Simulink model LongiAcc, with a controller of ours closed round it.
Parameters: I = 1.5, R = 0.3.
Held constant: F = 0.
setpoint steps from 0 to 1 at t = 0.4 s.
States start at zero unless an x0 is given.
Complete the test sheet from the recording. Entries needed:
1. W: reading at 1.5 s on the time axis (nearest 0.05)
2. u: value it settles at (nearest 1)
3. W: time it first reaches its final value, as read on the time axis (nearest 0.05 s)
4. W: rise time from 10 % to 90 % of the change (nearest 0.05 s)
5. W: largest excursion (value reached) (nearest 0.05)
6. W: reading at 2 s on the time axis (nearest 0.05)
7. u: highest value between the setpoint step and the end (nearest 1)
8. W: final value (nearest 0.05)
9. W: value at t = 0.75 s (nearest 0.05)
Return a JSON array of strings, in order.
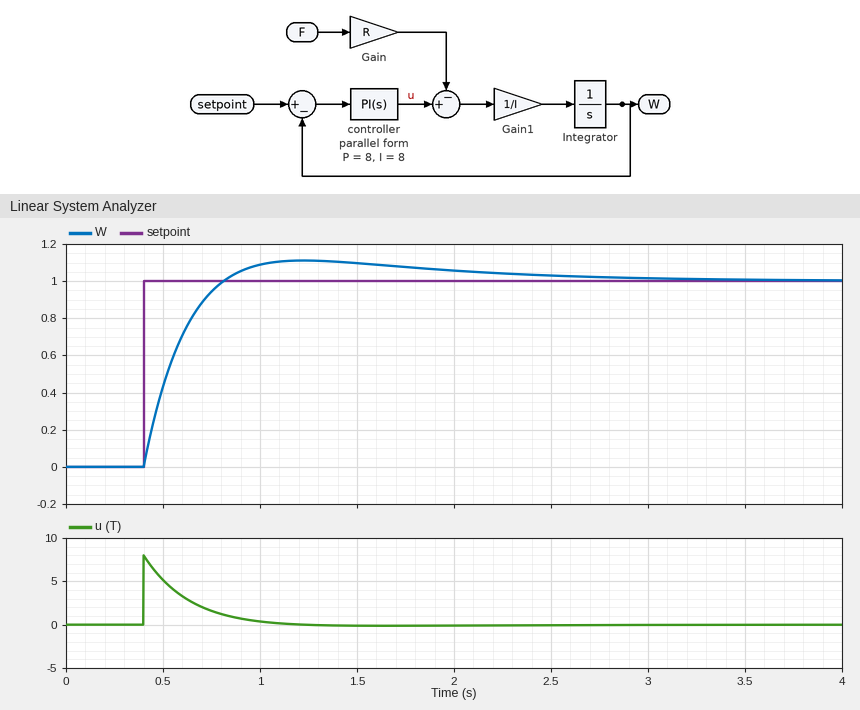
["1.10", "0", "0.80 s", "0.30 s", "1.10", "1.05", "8", "1.00", "0.95"]
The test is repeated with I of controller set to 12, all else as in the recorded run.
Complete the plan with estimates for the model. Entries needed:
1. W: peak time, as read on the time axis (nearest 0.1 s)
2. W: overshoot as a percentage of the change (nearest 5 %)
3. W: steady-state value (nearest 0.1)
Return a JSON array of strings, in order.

["1.1 s", "15 %", "1.0"]
